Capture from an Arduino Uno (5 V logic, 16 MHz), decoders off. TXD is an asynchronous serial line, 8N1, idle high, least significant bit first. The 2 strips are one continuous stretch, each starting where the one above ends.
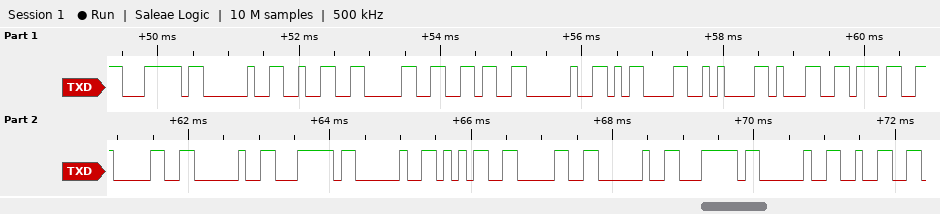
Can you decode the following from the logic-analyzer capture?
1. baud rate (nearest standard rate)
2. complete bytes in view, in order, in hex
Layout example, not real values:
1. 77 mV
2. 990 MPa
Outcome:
1. 9600 baud
2. 7C 20 32 30 36 20 0D 0A 31 37 30 20 7C 20 35 30 20 7C 20 32
